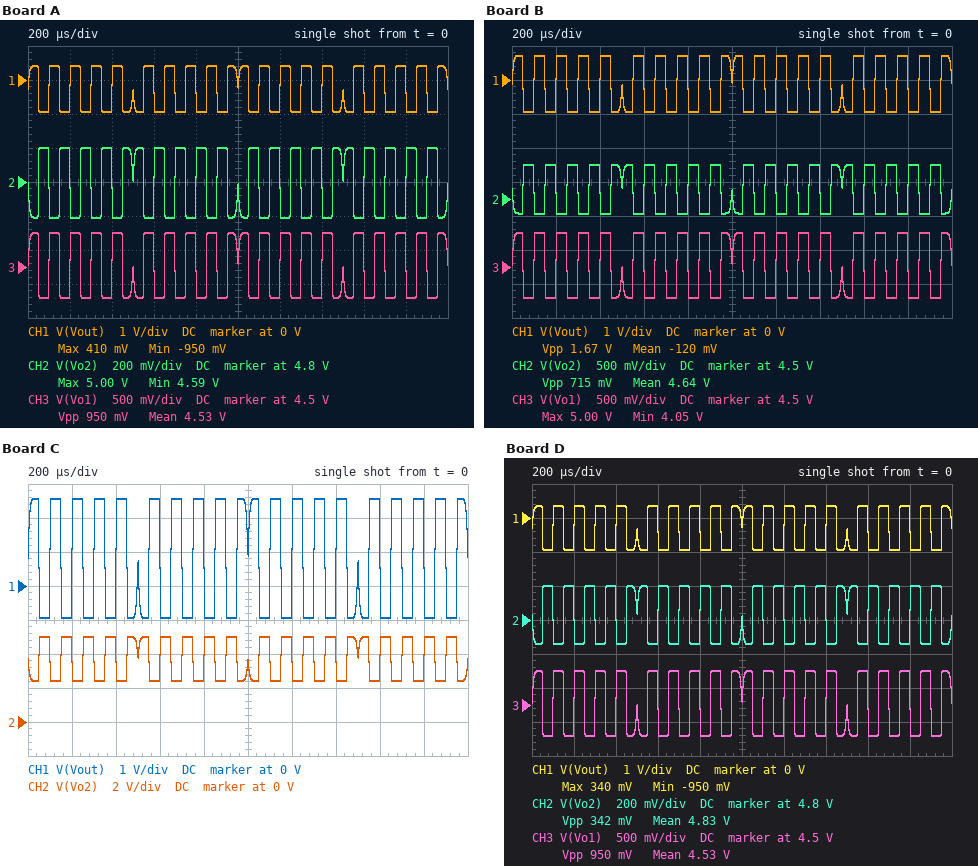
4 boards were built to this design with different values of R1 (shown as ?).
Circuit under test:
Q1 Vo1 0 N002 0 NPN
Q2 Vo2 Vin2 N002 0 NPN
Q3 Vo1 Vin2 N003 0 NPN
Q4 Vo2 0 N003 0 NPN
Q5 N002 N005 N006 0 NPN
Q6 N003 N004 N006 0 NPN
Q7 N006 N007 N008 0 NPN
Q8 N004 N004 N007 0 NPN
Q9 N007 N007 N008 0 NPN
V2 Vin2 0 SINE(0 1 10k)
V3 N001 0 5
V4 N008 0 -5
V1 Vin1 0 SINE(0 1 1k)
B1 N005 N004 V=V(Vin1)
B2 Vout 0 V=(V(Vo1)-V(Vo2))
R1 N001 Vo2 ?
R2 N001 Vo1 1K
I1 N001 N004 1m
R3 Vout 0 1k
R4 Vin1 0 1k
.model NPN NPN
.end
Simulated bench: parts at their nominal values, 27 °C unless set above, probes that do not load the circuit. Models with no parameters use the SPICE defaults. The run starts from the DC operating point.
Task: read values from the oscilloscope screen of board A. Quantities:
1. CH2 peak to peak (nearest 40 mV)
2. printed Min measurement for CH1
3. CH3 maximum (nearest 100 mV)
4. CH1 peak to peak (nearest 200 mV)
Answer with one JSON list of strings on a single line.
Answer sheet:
["400 mV", "-950 mV", "5.0 V", "1.4 V"]
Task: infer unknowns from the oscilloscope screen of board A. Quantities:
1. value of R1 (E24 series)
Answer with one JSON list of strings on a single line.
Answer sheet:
["430 Ω"]
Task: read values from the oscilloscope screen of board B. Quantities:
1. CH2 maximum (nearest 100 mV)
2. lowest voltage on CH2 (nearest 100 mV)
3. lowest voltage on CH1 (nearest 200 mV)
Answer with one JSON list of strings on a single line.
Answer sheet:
["5.0 V", "4.3 V", "-1.0 V"]
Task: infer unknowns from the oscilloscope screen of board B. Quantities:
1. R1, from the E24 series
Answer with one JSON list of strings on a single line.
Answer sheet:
["750 Ω"]
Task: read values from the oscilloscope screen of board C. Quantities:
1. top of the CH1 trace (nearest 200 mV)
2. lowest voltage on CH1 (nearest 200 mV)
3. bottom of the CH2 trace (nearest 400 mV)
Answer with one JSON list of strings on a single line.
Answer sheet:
["2.6 V", "-1.0 V", "2.4 V"]
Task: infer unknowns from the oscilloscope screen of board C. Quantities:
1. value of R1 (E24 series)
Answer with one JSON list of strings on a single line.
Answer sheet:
["2.7 kΩ"]
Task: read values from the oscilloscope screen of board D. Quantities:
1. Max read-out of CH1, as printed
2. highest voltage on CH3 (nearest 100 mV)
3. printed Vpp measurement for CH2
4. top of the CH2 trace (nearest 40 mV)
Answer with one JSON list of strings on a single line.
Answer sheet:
["340 mV", "5.0 V", "342 mV", "5.00 V"]
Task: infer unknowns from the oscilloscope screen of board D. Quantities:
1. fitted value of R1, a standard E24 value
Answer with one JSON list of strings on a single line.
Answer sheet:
["360 Ω"]
